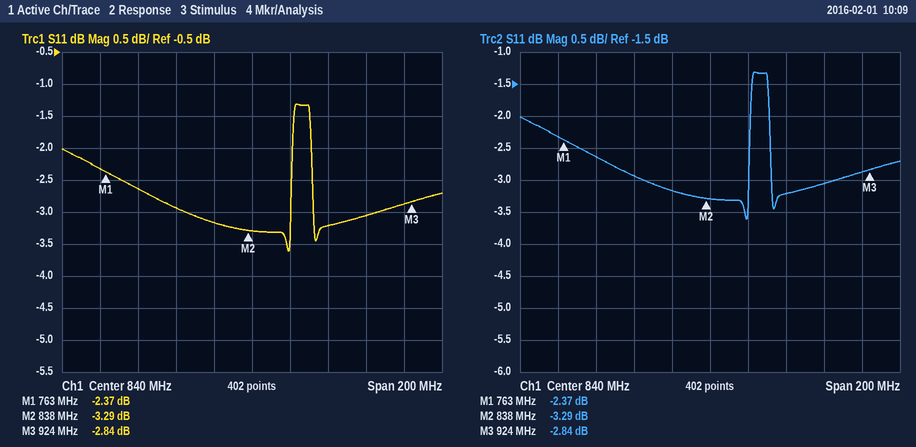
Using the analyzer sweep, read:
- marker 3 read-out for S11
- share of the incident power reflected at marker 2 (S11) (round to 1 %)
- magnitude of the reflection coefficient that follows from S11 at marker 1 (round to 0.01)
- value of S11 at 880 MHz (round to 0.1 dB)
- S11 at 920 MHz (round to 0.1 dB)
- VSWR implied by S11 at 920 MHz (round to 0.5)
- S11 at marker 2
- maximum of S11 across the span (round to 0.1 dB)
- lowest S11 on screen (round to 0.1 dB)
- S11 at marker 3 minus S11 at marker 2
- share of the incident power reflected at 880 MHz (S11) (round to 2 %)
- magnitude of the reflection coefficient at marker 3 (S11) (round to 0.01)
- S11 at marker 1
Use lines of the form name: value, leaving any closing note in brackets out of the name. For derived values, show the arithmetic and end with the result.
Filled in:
marker 3 read-out for S11: -2.84 dB
share of the incident power reflected at marker 2 (S11): 10^(-3.29/10) ≈ 47 %
magnitude of the reflection coefficient that follows from S11 at marker 1: 10^(-2.37/20) ≈ 0.76
value of S11 at 880 MHz: -3.2 dB
S11 at 920 MHz: -2.9 dB
VSWR implied by S11 at 920 MHz: |Γ| = 10^(-2.9/20) = 0.7161; VSWR = (1 + 0.7161)/(1 − 0.7161) ≈ 6.0
S11 at marker 2: -3.29 dB
maximum of S11 across the span: -1.3 dB
lowest S11 on screen: -3.6 dB
S11 at marker 3 minus S11 at marker 2: -2.84 − (-3.29) = 0.45 dB
share of the incident power reflected at 880 MHz (S11): 10^(-3.2/10) ≈ 48 %
magnitude of the reflection coefficient at marker 3 (S11): 10^(-2.84/20) ≈ 0.72
S11 at marker 1: -2.37 dB
